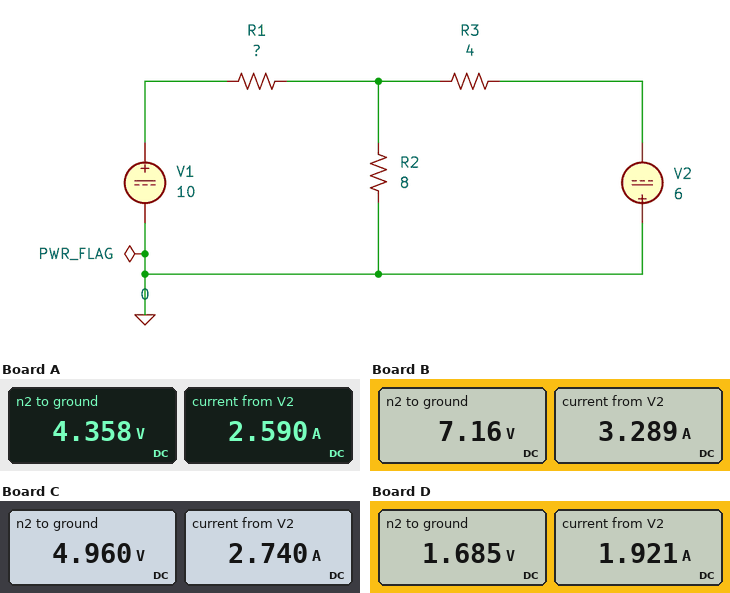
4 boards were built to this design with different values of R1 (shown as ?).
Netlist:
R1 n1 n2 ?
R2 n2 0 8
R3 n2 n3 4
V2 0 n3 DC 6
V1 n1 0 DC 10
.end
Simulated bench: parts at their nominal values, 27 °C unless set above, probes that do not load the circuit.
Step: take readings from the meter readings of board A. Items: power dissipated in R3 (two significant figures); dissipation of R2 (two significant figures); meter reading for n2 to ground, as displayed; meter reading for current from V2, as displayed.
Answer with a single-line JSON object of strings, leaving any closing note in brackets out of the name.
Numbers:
{"power dissipated in R3": "27 W", "dissipation of R2": "2.4 W", "meter reading for n2 to ground, as displayed": "4.358 V", "meter reading for current from V2, as displayed": "2.590 A"}
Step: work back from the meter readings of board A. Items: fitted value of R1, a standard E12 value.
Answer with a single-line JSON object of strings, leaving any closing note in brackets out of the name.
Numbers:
{"fitted value of R1, a standard E12 value": "1.8 Ω"}
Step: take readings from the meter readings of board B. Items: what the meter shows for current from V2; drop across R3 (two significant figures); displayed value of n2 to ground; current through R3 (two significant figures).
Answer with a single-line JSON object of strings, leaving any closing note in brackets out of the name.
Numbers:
{"what the meter shows for current from V2": "3.289 A", "drop across R3": "13 V", "displayed value of n2 to ground": "7.16 V", "current through R3": "3.3 A"}
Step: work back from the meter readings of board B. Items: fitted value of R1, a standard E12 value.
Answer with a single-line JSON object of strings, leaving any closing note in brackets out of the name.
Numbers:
{"fitted value of R1, a standard E12 value": "0.68 Ω"}
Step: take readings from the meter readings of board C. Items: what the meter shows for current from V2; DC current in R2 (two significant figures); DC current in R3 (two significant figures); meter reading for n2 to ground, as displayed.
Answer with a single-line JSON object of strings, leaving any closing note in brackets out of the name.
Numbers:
{"what the meter shows for current from V2": "2.740 A", "DC current in R2": "620 mA", "DC current in R3": "2.7 A", "meter reading for n2 to ground, as displayed": "4.960 V"}
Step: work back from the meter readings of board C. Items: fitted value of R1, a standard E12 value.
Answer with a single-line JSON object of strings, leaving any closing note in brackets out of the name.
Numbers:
{"fitted value of R1, a standard E12 value": "1.5 Ω"}
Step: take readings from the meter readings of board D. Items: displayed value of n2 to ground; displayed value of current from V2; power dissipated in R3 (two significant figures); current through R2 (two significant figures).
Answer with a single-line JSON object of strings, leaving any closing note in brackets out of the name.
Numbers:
{"displayed value of n2 to ground": "1.685 V", "displayed value of current from V2": "1.921 A", "power dissipated in R3": "15 W", "current through R2": "210 mA"}
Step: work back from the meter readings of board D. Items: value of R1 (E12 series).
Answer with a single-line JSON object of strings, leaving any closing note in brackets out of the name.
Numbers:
{"value of R1": "3.9 Ω"}
